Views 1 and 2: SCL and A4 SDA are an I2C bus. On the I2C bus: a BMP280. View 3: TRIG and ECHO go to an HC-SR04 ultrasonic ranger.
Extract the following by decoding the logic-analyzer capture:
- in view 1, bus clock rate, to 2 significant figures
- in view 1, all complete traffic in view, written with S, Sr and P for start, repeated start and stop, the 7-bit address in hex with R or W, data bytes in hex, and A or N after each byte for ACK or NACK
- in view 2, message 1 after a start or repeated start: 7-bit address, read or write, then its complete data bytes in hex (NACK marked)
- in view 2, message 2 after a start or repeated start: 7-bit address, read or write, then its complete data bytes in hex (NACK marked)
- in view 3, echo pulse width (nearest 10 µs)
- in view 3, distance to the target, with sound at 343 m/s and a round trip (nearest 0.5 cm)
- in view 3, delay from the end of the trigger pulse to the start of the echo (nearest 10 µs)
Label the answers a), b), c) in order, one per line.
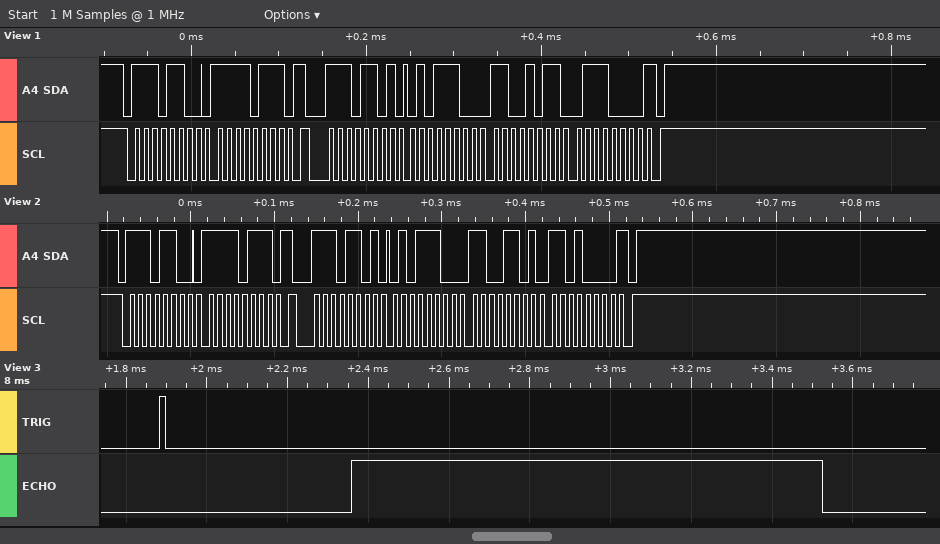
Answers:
a) 100 kHz
b) S 76W A F7 A Sr 76R A 5C A CB A 70 N P
c) 0x76 write: F7
d) 0x76 read: 5C CD D0 NACK
e) 1170 µs
f) 20 cm
g) 460 µs
